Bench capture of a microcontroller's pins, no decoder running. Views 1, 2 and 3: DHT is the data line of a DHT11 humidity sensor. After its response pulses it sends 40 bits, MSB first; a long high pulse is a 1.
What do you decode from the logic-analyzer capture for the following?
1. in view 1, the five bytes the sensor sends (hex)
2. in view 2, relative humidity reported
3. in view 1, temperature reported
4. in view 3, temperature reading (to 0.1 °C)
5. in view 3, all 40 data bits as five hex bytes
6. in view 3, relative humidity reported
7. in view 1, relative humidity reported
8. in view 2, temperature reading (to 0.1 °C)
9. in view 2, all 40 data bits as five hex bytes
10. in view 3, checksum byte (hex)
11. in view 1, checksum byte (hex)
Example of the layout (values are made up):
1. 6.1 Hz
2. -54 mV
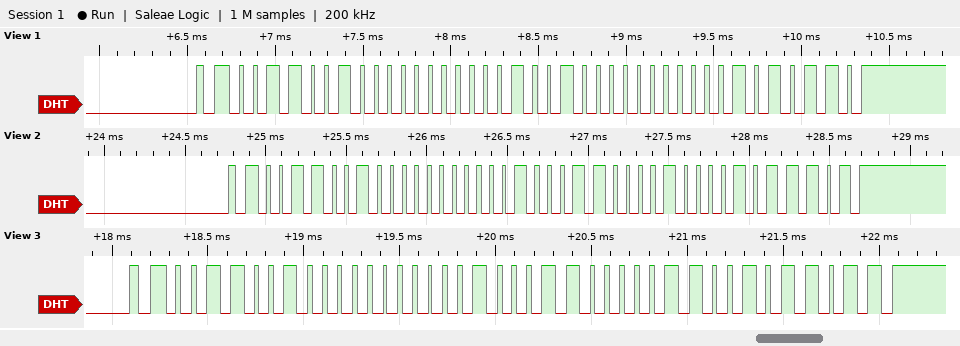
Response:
1. 32 00 24 00 56
2. 50 %
3. 36.0 °C
4. 35.6 °C
5. 32 00 23 06 5B
6. 50 %
7. 50 %
8. 35.8 °C
9. 32 00 23 08 5D
10. 0x5B
11. 0x56
